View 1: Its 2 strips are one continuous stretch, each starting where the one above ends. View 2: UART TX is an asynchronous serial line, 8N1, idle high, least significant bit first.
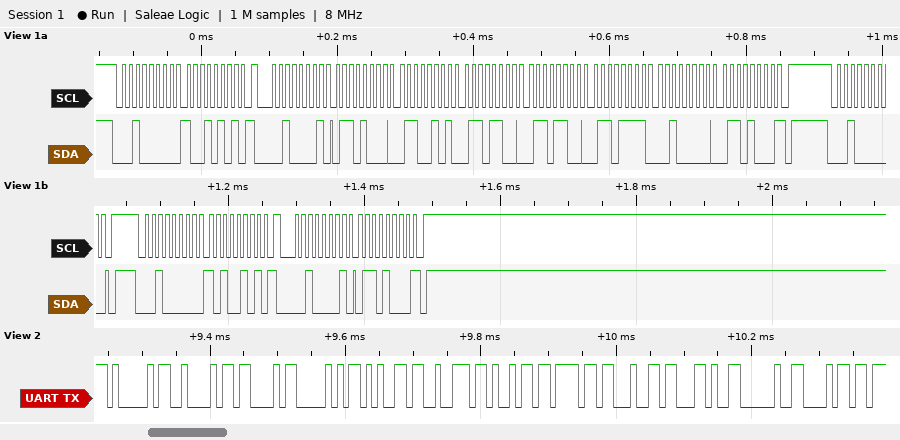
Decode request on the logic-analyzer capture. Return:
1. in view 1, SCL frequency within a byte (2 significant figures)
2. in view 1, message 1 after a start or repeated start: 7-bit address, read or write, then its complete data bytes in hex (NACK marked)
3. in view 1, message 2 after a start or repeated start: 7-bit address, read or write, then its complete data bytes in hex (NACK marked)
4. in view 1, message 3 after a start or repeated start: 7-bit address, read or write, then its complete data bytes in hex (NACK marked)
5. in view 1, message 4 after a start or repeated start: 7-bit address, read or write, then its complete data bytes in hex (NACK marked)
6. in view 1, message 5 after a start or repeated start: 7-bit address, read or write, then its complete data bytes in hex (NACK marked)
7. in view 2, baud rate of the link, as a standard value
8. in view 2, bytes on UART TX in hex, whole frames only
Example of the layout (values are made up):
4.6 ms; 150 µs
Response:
100 kHz; 0x10 write: 95; 0x10 read: 68 65 6C 6C 6F 20 68 NACK; 0x10 write; 0x10 write: A5; 0x10 read: 68 NACK; 115200 baud; 41 42 43 50 65 72 69 6F 64 2C 20 68
